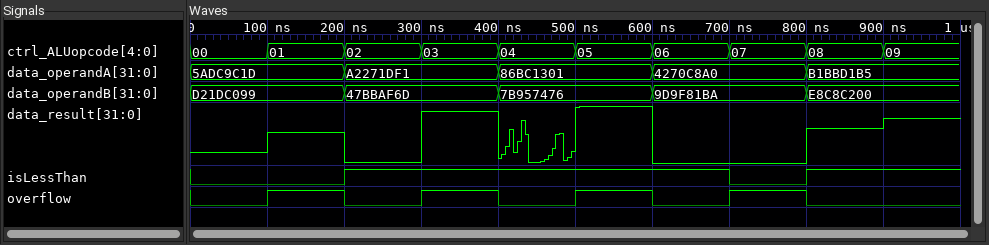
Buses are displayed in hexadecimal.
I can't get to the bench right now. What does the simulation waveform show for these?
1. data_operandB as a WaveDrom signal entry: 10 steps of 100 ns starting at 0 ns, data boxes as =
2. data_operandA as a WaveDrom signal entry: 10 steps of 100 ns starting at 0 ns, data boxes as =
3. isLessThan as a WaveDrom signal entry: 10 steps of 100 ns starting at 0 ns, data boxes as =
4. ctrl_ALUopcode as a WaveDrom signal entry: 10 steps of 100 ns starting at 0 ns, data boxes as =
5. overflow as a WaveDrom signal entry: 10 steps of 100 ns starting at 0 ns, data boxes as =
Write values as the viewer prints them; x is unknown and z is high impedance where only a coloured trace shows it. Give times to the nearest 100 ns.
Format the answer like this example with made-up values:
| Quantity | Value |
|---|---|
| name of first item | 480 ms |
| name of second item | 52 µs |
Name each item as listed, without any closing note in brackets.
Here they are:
| Quantity | Value |
|---|---|
| data_operandB as a WaveDrom signal entry: 10 steps of 100 ns starting at 0 ns, data boxes as = | {name: 'data_operandB', wave: '=.=.=.=.=.', data: 'D21DC099 47BBAF6D 7B957476 9D9F81BA E8C8C200'} |
| data_operandA as a WaveDrom signal entry: 10 steps of 100 ns starting at 0 ns, data boxes as = | {name: 'data_operandA', wave: '=.=.=.=.=.', data: '5ADC9C1D A2271DF1 86BC1301 4270C8A0 B1BBD1B5'} |
| isLessThan as a WaveDrom signal entry: 10 steps of 100 ns starting at 0 ns, data boxes as = | {name: 'isLessThan', wave: '0.1....01.'} |
| ctrl_ALUopcode as a WaveDrom signal entry: 10 steps of 100 ns starting at 0 ns, data boxes as = | {name: 'ctrl_ALUopcode', wave: '==========', data: '00 01 02 03 04 05 06 07 08 09'} |
| overflow as a WaveDrom signal entry: 10 steps of 100 ns starting at 0 ns, data boxes as = | {name: 'overflow', wave: '010101010.'} |
